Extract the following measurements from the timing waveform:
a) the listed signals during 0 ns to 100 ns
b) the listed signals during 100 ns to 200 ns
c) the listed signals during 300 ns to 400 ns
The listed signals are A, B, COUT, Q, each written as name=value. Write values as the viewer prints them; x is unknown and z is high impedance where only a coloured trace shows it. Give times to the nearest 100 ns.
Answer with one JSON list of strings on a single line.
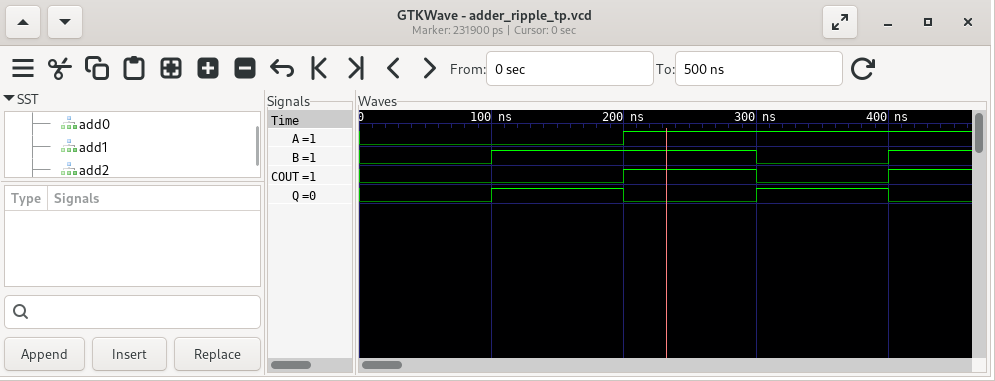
["A=0, B=0, COUT=0, Q=0", "A=0, B=1, COUT=0, Q=1", "A=1, B=0, COUT=0, Q=1"]
